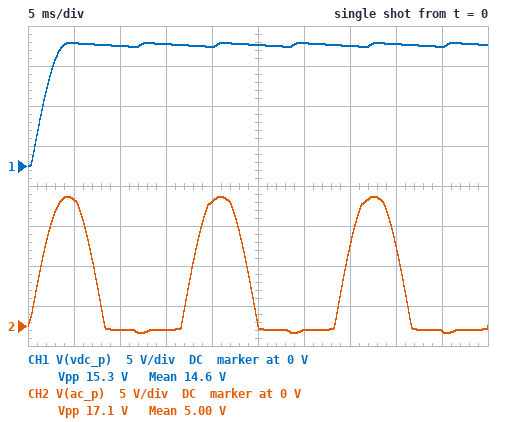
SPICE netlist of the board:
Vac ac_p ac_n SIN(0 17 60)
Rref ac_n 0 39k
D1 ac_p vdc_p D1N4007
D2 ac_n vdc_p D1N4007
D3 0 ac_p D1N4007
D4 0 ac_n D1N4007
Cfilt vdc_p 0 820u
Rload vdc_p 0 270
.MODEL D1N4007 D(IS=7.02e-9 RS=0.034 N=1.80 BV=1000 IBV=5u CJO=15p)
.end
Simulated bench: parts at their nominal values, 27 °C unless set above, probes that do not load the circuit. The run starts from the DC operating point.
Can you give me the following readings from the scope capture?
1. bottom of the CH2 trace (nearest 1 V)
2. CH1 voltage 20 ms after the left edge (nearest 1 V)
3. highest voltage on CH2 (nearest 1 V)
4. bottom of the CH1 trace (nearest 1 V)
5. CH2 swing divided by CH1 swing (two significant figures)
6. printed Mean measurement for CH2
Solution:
-1 V
15 V
16 V
0 V
1.1
5.00 V
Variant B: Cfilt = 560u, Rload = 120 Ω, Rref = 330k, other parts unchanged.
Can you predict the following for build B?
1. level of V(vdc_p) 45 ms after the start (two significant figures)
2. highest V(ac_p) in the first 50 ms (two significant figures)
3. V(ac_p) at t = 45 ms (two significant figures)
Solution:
14 V
16 V
-930 mV
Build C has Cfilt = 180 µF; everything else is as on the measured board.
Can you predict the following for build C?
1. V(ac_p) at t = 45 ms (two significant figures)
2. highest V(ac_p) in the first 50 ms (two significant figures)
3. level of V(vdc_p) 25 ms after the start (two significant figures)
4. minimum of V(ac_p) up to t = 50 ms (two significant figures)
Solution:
-850 mV
16 V
14 V
-860 mV
